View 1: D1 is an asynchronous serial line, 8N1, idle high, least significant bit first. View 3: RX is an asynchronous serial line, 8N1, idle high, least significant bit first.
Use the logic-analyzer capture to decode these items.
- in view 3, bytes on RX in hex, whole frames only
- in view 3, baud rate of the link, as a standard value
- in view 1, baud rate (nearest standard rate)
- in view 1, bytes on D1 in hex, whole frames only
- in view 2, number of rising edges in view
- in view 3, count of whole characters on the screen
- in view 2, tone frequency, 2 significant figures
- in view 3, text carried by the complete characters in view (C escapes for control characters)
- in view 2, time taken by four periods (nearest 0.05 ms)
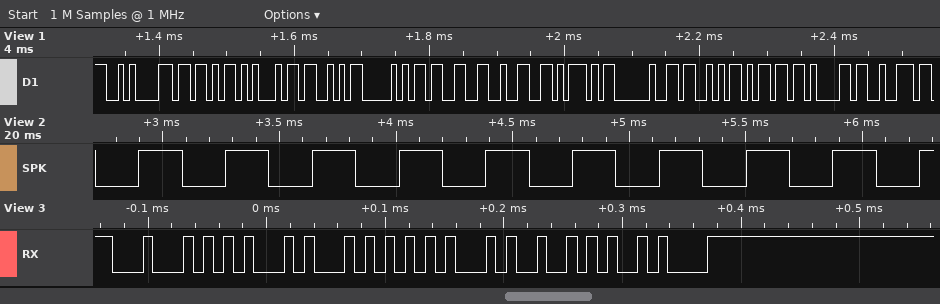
44 45 54 45 52 0A
115200 baud
115200 baud
0A 5B 45 53 50 33 32 5D 20 53 6D 61 72
10
6
2.7 kHz
"DETER\n"
1.50 ms
